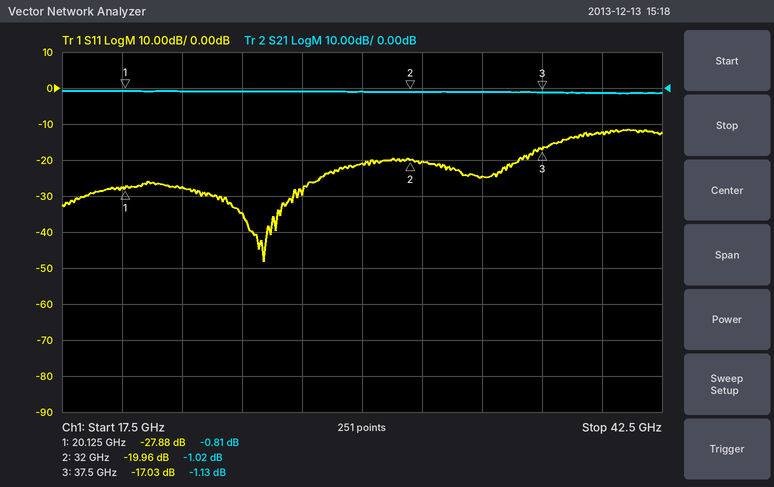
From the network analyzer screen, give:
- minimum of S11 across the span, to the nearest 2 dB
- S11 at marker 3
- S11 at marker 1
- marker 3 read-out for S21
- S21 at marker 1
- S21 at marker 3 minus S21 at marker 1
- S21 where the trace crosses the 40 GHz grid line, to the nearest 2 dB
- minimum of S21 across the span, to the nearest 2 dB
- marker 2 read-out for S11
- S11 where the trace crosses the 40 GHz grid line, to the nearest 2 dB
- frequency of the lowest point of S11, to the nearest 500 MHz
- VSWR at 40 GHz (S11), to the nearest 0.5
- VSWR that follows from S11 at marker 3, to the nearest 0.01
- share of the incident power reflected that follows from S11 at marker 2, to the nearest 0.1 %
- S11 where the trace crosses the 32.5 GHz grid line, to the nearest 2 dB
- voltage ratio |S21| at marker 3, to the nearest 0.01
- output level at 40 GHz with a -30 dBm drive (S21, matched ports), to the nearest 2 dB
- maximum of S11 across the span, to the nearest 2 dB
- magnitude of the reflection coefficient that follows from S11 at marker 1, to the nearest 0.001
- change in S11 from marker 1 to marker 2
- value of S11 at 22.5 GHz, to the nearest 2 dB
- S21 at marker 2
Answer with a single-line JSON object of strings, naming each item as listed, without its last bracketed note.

{"minimum of S11 across the span, to the nearest 2 dB": "-48 dB", "S11 at marker 3": "-17.03 dB", "S11 at marker 1": "-27.88 dB", "marker 3 read-out for S21": "-1.13 dB", "S21 at marker 1": "-0.81 dB", "S21 at marker 3 minus S21 at marker 1": "-0.32 dB", "S21 where the trace crosses the 40 GHz grid line, to the nearest 2 dB": "-2 dB", "minimum of S21 across the span, to the nearest 2 dB": "-2 dB", "marker 2 read-out for S11": "-19.96 dB", "S11 where the trace crosses the 40 GHz grid line, to the nearest 2 dB": "-12 dB", "frequency of the lowest point of S11, to the nearest 500 MHz": "26.0 GHz", "VSWR at 40 GHz (S11), to the nearest 0.5": "1.5", "VSWR that follows from S11 at marker 3, to the nearest 0.01": "1.33", "share of the incident power reflected that follows from S11 at marker 2, to the nearest 0.1 %": "1.0 %", "S11 where the trace crosses the 32.5 GHz grid line, to the nearest 2 dB": "-20 dB", "voltage ratio |S21| at marker 3, to the nearest 0.01": "0.88", "output level at 40 GHz with a -30 dBm drive (S21, matched ports), to the nearest 2 dB": "-32 dBm", "maximum of S11 across the span, to the nearest 2 dB": "-12 dB", "magnitude of the reflection coefficient that follows from S11 at marker 1, to the nearest 0.001": "0.040", "change in S11 from marker 1 to marker 2": "7.92 dB", "value of S11 at 22.5 GHz, to the nearest 2 dB": "-28 dB", "S21 at marker 2": "-1.02 dB"}
